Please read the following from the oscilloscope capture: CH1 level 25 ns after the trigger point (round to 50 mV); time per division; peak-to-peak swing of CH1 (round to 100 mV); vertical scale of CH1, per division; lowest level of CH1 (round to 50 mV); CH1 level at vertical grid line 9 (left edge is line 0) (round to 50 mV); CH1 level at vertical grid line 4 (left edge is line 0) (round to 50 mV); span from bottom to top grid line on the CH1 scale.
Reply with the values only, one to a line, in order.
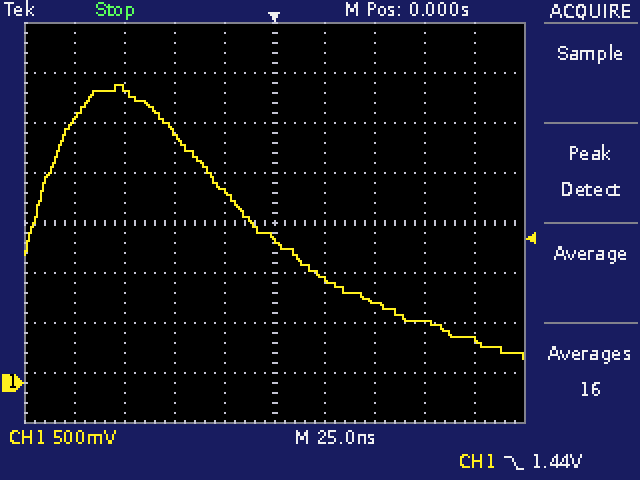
1.05 V
25 ns
2.70 V
500 mV
250 mV
450 mV
1.90 V
4 V
